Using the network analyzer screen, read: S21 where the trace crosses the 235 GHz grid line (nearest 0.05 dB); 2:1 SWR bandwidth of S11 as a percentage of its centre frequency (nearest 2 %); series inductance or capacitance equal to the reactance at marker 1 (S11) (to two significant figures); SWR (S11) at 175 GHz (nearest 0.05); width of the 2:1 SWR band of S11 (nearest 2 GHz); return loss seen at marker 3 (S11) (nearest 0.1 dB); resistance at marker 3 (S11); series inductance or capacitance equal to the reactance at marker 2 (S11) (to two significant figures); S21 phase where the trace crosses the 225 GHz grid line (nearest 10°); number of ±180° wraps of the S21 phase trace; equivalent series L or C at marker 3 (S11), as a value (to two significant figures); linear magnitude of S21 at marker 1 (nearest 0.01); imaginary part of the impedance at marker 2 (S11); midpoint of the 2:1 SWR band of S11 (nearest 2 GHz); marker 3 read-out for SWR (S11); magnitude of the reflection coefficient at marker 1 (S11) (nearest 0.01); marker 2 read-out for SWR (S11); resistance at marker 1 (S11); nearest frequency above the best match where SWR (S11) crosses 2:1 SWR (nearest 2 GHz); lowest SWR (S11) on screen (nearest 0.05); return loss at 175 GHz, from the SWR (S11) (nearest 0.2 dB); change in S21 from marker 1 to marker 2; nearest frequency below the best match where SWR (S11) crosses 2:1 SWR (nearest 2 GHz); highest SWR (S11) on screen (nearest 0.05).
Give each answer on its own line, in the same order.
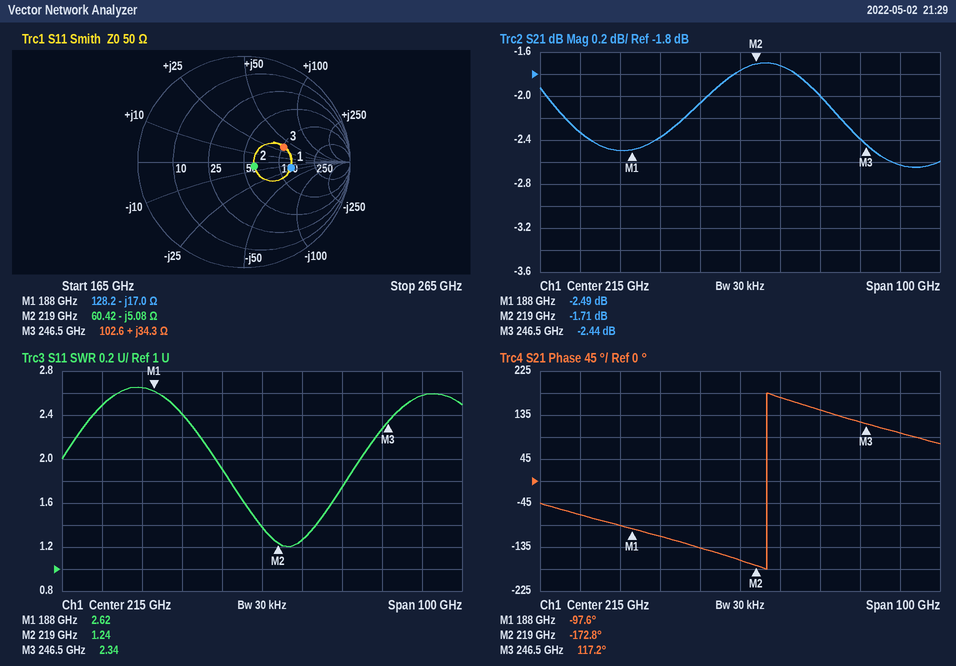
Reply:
-2.00 dB
16 %
50 fF
2.50
36 GHz
7.9 dB
102.6 Ω
140 fF
170°
1
22 pH
0.75
-5.08 Ω
222 GHz
2.34
0.45
1.24
128.2 Ω
240 GHz
1.20
7.4 dB
0.78 dB
204 GHz
2.65
